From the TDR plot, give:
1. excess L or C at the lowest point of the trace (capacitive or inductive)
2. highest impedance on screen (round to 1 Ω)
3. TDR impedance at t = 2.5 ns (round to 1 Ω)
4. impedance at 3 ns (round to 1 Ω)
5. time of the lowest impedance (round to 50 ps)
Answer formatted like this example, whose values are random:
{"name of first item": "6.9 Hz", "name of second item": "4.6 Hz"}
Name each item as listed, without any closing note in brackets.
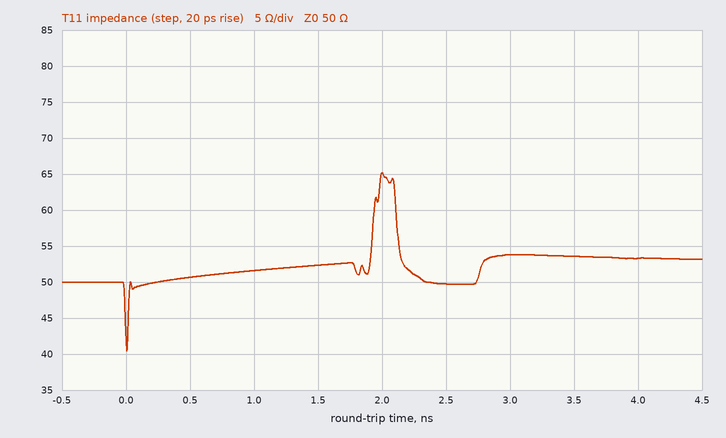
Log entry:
{"excess L or C at the lowest point of the trace": "capacitive", "highest impedance on screen": "65 Ω", "TDR impedance at t = 2.5 ns": "50 Ω", "impedance at 3 ns": "54 Ω", "time of the lowest impedance": "0 ps"}
